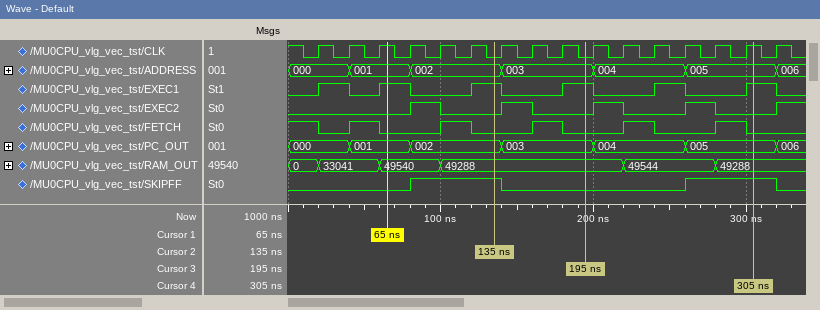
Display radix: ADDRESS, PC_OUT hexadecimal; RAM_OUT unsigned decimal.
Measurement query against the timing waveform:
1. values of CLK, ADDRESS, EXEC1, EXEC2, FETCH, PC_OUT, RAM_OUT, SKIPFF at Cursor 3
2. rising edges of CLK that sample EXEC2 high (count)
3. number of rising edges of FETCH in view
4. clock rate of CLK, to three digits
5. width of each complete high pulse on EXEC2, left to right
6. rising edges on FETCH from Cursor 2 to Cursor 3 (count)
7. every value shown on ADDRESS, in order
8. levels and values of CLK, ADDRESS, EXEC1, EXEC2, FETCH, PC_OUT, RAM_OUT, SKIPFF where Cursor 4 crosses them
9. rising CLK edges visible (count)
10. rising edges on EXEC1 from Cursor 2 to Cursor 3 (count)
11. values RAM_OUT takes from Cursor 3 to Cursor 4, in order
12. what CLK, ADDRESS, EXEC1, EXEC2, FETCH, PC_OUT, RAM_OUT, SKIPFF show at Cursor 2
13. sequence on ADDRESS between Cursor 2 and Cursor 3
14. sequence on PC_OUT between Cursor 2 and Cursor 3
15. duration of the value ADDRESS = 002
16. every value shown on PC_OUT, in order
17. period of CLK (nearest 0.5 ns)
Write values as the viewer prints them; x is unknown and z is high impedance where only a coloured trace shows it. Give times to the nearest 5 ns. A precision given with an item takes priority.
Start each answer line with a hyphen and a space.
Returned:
- CLK=0, ADDRESS=003, EXEC1=1, EXEC2=0, FETCH=0, PC_OUT=003, RAM_OUT=49288, SKIPFF=0
- 4
- 5
- 50.0 MHz
- 20 ns, 20 ns, 20 ns, 20 ns
- 1
- 000, 001, 002, 003, 004, 005, 006
- CLK=1, ADDRESS=005, EXEC1=1, EXEC2=0, FETCH=0, PC_OUT=005, RAM_OUT=49288, SKIPFF=1
- 16
- 1
- 49288, 49544, 49288
- CLK=0, ADDRESS=002, EXEC1=1, EXEC2=0, FETCH=0, PC_OUT=002, RAM_OUT=49288, SKIPFF=1
- 002, 003
- 002, 003
- 60 ns
- 000, 001, 002, 003, 004, 005, 006
- 20 ns
